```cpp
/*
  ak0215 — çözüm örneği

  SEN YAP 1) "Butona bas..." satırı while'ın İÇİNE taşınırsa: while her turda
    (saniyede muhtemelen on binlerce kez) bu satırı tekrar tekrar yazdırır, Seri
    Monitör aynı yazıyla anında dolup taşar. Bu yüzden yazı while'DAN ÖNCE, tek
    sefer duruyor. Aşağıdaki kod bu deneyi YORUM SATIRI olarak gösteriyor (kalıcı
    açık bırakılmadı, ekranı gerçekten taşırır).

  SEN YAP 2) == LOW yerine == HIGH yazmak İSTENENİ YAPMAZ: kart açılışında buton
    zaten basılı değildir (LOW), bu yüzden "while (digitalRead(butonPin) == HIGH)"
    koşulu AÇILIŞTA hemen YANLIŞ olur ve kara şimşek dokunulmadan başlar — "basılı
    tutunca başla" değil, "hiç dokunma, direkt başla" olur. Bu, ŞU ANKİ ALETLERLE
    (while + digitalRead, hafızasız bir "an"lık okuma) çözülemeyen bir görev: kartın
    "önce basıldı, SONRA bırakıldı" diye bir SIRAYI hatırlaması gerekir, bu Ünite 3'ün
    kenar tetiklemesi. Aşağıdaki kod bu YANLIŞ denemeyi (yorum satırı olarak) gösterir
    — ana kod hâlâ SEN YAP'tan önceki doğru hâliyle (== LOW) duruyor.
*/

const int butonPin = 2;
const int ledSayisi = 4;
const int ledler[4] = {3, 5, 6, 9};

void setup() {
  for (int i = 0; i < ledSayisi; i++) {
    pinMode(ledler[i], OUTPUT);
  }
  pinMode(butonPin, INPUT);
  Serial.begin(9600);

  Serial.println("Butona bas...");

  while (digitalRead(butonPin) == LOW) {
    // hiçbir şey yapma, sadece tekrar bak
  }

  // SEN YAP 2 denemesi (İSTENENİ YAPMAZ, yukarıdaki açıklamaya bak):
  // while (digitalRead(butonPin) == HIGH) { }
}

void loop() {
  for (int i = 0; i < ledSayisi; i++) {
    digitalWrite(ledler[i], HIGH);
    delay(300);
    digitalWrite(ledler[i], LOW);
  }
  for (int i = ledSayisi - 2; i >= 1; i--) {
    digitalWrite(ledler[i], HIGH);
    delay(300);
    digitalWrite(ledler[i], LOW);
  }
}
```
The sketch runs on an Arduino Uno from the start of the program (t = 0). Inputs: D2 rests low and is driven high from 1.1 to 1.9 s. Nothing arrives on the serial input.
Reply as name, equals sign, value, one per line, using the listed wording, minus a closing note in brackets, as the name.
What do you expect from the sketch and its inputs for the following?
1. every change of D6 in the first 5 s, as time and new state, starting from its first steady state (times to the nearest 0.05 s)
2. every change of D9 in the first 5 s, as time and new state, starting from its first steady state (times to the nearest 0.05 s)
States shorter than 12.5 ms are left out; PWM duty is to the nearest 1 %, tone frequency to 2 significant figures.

every change of D6 in the first 5 s, as time and new state, starting from its first steady state = 0 s low; 1.7 s high; 2 s low; 2.3 s high; 2.6 s low; 3.5 s high; 3.8 s low; 4.1 s high; 4.4 s low
every change of D9 in the first 5 s, as time and new state, starting from its first steady state = 0 s low; 2 s high; 2.3 s low; 3.8 s high; 4.1 s low
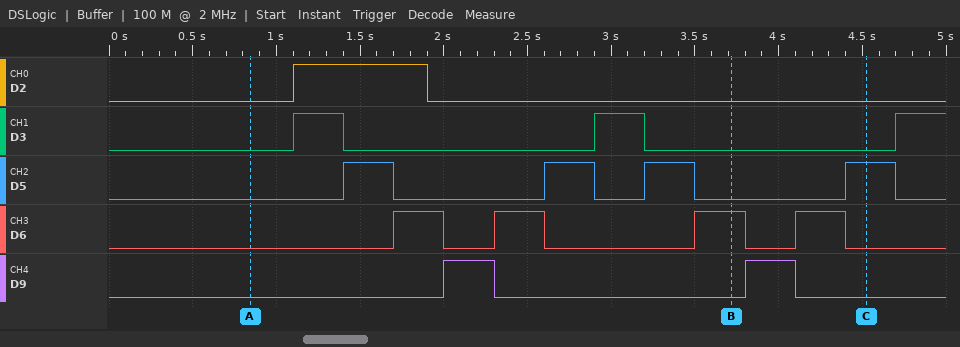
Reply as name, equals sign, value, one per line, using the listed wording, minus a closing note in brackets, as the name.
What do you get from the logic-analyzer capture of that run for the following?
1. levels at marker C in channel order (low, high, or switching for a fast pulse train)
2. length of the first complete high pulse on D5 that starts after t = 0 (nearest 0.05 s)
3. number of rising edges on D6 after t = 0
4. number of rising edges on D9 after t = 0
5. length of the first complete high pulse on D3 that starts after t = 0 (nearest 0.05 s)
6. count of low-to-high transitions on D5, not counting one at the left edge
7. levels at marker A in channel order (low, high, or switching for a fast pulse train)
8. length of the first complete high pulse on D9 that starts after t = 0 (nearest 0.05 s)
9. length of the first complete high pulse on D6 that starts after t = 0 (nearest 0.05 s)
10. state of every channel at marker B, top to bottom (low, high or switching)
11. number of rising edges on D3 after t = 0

levels at marker C in channel order = D2 low, D3 low, D5 high, D6 low, D9 low
length of the first complete high pulse on D5 that starts after t = 0 = 0.30 s
number of rising edges on D6 after t = 0 = 4
number of rising edges on D9 after t = 0 = 2
length of the first complete high pulse on D3 that starts after t = 0 = 0.30 s
count of low-to-high transitions on D5, not counting one at the left edge = 4
levels at marker A in channel order = D2 low, D3 low, D5 low, D6 low, D9 low
length of the first complete high pulse on D9 that starts after t = 0 = 0.30 s
length of the first complete high pulse on D6 that starts after t = 0 = 0.30 s
state of every channel at marker B, top to bottom = D2 low, D3 low, D5 low, D6 high, D9 low
number of rising edges on D3 after t = 0 = 3
